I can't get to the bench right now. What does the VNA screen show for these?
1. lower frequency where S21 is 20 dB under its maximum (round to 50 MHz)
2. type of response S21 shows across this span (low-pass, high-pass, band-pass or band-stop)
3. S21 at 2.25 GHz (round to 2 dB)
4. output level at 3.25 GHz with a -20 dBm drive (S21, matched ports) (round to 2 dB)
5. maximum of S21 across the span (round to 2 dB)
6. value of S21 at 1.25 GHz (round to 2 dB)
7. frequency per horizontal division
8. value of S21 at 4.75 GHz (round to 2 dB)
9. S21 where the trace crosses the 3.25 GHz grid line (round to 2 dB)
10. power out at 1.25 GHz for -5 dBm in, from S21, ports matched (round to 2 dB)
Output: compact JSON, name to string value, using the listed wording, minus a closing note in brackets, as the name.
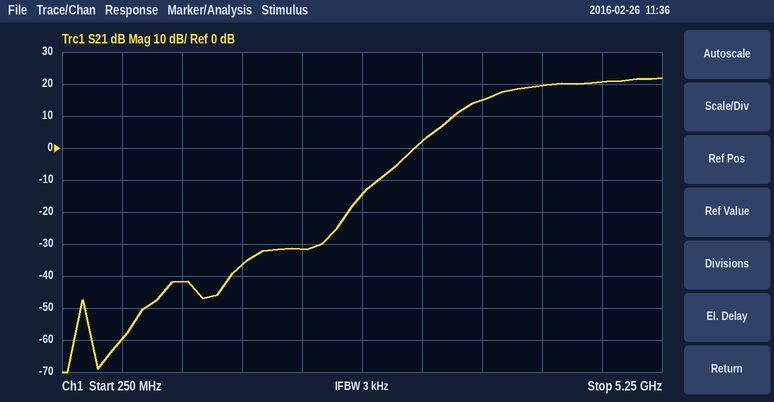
{"lower frequency where S21 is 20 dB under its maximum": "3.25 GHz", "type of response S21 shows across this span": "high-pass", "S21 at 2.25 GHz": "-32 dB", "output level at 3.25 GHz with a -20 dBm drive (S21, matched ports)": "-18 dBm", "maximum of S21 across the span": "22 dB", "value of S21 at 1.25 GHz": "-42 dB", "frequency per horizontal division": "500 MHz", "value of S21 at 4.75 GHz": "20 dB", "S21 where the trace crosses the 3.25 GHz grid line": "2 dB", "power out at 1.25 GHz for -5 dBm in, from S21, ports matched": "-46 dBm"}
